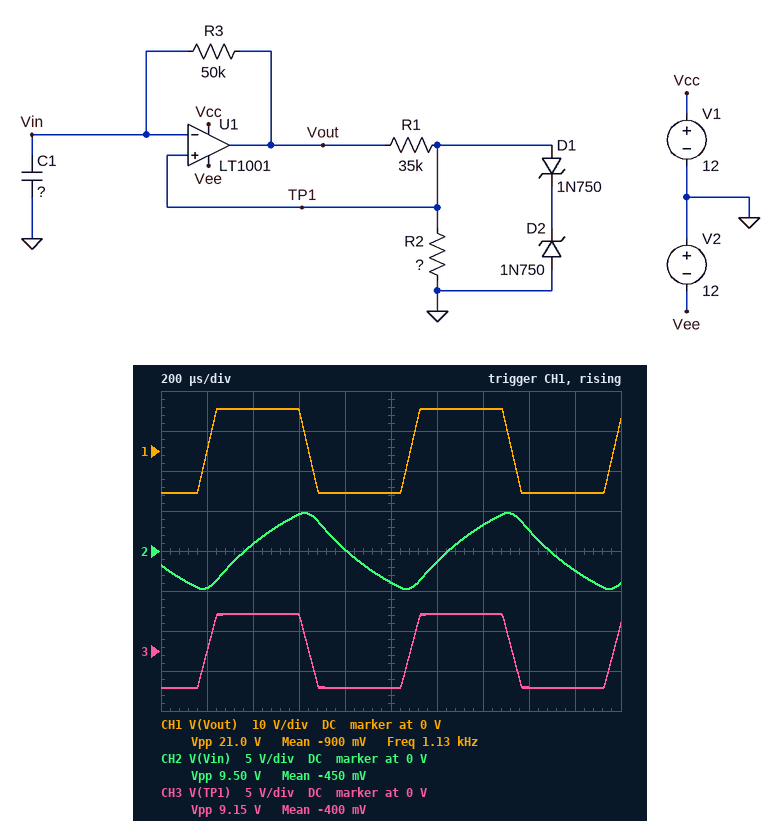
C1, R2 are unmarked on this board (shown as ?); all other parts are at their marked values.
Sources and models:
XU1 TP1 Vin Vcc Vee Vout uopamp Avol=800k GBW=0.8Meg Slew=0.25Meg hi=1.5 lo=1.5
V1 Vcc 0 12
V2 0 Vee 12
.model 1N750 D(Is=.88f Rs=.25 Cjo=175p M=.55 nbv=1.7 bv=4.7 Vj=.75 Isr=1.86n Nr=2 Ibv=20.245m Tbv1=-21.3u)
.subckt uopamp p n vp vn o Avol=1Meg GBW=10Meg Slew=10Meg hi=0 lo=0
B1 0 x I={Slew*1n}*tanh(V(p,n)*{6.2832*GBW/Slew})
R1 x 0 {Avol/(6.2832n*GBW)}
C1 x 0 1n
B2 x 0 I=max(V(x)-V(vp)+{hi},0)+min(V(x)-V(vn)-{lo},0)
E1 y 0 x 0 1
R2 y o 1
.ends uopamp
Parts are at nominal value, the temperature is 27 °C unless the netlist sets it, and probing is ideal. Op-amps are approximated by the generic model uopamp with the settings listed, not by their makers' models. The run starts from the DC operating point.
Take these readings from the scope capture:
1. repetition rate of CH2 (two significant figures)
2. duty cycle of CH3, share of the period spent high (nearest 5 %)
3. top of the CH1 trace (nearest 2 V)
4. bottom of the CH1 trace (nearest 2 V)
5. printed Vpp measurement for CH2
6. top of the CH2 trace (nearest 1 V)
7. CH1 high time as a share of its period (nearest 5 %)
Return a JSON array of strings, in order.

["1.1 kHz", "50 %", "10 V", "-10 V", "9.50 V", "5 V", "50 %"]
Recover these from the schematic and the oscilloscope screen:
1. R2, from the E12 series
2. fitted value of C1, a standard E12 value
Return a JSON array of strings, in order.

["27 kΩ", "8.2 nF"]
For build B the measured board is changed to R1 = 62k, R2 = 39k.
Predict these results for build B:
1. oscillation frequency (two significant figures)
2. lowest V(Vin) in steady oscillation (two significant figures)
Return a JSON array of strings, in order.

["1.3 kHz", "-4.3 V"]
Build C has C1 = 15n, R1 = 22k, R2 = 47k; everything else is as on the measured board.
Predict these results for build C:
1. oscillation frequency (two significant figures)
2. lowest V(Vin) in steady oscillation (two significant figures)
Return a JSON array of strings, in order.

["580 Hz", "-5.2 V"]
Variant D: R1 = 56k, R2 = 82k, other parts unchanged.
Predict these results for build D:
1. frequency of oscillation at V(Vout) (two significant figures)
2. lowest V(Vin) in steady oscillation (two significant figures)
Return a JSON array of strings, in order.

["1.0 kHz", "-5.1 V"]
